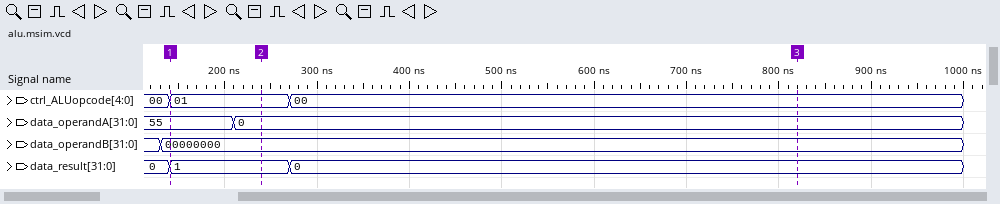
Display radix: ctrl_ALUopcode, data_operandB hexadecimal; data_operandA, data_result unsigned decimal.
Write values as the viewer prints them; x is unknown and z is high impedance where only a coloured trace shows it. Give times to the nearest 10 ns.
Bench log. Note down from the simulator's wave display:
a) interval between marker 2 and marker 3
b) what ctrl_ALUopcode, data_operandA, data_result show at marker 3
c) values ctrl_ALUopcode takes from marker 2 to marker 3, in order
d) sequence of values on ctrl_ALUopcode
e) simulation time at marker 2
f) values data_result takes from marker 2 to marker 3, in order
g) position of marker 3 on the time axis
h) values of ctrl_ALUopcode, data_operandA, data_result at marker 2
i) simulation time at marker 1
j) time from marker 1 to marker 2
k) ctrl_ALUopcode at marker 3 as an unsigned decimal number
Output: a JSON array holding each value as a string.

["580 ns", "ctrl_ALUopcode=00, data_operandA=0, data_result=0", "01, 00", "00, 01, 00", "240 ns", "1, 0", "820 ns", "ctrl_ALUopcode=01, data_operandA=0, data_result=1", "140 ns", "100 ns", "0"]
